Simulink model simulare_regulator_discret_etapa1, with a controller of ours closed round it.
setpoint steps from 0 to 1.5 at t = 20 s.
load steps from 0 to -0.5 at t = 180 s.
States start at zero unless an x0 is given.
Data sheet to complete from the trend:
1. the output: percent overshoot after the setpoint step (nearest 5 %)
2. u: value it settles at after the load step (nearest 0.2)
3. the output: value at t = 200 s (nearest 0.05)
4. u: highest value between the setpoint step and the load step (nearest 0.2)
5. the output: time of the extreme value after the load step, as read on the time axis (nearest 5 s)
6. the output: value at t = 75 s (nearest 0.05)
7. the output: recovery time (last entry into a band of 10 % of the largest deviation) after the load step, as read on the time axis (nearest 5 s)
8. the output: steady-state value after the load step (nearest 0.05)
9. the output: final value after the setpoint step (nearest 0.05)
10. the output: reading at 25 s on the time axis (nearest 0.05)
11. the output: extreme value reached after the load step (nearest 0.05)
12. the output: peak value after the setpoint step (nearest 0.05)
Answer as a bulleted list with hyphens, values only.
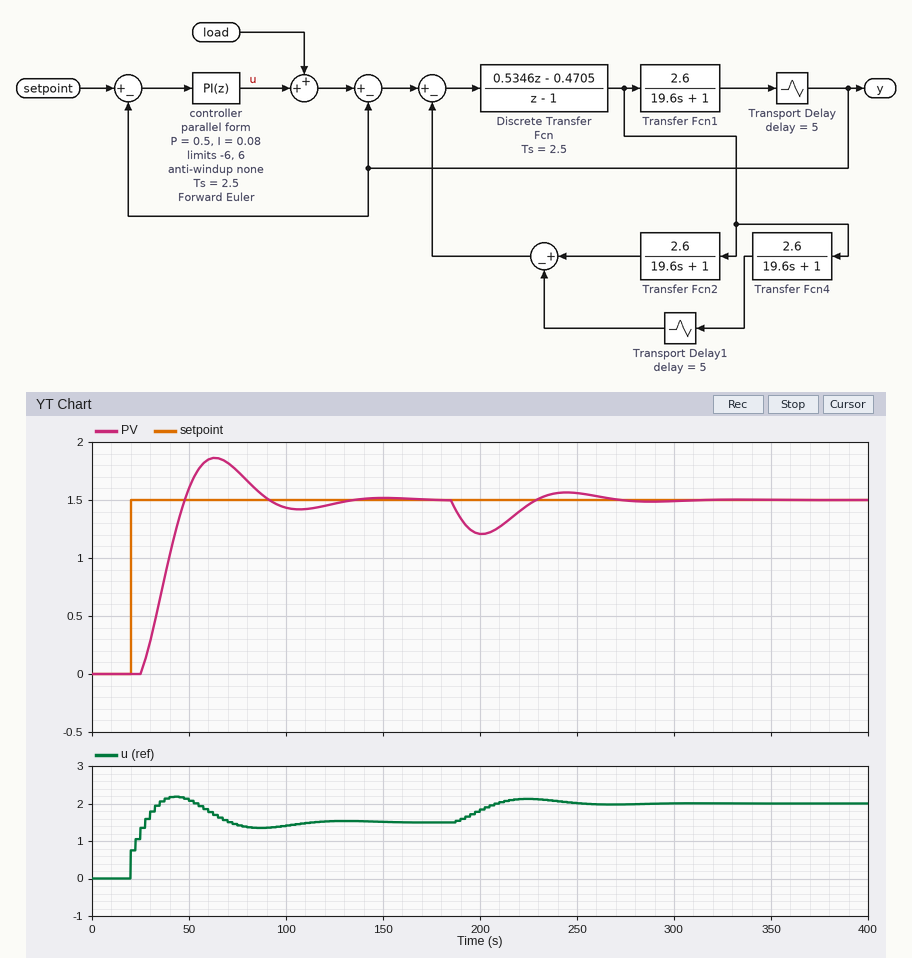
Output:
- 25 %
- 2.0
- 1.20
- 2.2
- 200 s
- 1.75
- 260 s
- 1.50
- 1.50
- 0.00
- 1.20
- 1.85
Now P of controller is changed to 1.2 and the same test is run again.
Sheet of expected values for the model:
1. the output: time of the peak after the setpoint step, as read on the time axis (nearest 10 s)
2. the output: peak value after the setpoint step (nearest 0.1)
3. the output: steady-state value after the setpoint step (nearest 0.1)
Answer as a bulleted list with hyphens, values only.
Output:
- 50 s
- 1.6
- 1.5
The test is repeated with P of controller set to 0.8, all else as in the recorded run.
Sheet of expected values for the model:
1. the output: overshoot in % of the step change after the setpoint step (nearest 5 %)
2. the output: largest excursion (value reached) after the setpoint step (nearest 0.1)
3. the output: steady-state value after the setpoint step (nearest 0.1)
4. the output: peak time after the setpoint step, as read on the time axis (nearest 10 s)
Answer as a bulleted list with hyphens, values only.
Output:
- 15 %
- 1.7
- 1.5
- 60 s
